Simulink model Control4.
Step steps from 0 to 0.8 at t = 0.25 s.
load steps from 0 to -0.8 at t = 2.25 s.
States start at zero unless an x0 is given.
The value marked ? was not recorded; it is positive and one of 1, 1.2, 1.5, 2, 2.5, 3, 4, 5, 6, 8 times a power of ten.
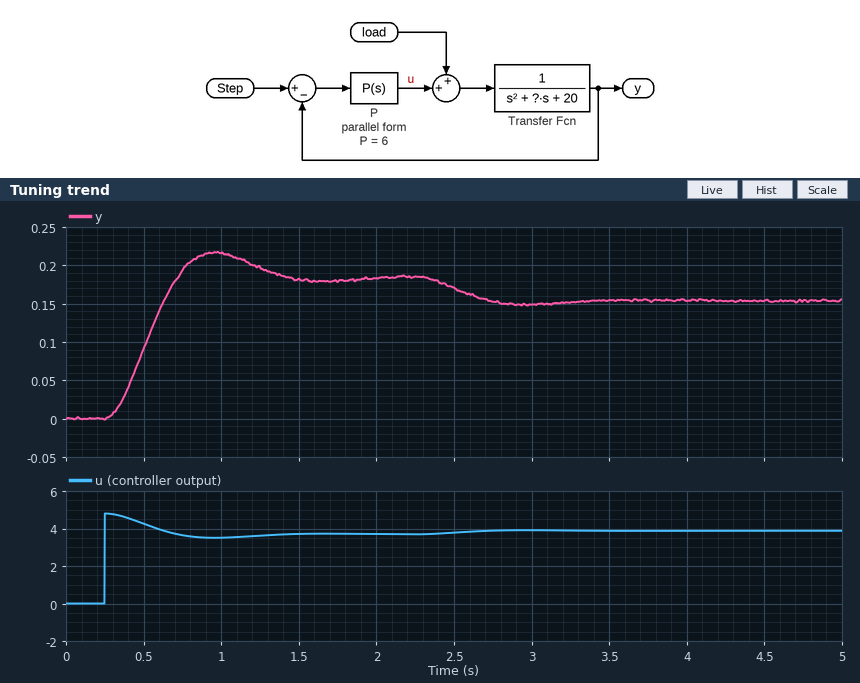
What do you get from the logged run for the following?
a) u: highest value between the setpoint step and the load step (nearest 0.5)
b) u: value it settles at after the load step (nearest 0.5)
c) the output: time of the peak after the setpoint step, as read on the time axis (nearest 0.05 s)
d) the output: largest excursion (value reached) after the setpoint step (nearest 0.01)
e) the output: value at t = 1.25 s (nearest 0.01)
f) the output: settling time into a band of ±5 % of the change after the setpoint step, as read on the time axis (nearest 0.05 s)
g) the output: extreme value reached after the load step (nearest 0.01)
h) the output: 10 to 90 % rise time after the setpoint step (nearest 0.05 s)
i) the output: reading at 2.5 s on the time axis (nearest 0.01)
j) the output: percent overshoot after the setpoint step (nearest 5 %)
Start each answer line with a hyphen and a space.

- 5.0
- 4.0
- 0.95 s
- 0.22
- 0.20
- 1.30 s
- 0.15
- 0.30 s
- 0.17
- 15 %
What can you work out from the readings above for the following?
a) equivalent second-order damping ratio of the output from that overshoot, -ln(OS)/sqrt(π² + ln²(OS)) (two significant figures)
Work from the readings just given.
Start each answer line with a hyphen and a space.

- 0.52
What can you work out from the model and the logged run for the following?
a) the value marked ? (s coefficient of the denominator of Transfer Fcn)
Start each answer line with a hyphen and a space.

- 5
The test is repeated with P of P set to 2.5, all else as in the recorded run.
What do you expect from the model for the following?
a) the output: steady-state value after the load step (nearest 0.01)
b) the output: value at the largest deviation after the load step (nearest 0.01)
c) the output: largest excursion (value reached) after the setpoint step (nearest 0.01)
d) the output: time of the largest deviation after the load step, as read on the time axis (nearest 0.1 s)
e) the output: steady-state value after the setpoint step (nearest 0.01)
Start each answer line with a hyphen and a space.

- 0.05
- 0.05
- 0.10
- 3.0 s
- 0.09
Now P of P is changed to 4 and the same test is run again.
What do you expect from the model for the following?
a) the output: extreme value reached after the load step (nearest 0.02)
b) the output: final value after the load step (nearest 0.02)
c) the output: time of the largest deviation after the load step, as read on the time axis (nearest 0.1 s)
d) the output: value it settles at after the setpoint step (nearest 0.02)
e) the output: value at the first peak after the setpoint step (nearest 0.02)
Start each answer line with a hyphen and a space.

- 0.10
- 0.10
- 3.0 s
- 0.14
- 0.16
